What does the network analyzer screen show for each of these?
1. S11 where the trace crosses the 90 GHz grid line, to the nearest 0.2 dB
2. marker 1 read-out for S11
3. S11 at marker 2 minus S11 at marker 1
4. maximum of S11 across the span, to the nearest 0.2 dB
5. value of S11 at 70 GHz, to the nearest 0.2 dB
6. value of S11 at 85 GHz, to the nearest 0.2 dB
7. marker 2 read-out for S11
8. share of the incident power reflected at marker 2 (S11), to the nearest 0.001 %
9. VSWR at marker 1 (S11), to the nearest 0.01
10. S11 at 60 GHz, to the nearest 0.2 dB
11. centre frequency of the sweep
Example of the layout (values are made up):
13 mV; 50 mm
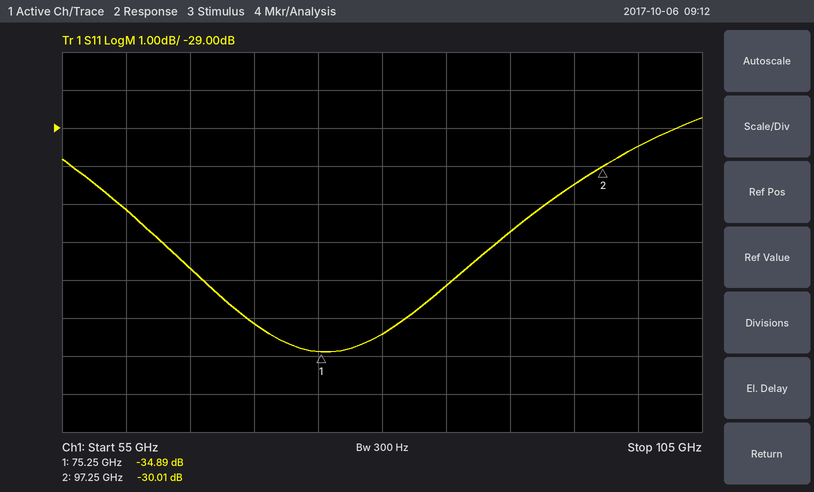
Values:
-31.8 dB; -34.89 dB; 4.88 dB; -28.8 dB; -34.2 dB; -33.2 dB; -30.01 dB; 0.100 %; 1.04; -31.2 dB; 80 GHz
